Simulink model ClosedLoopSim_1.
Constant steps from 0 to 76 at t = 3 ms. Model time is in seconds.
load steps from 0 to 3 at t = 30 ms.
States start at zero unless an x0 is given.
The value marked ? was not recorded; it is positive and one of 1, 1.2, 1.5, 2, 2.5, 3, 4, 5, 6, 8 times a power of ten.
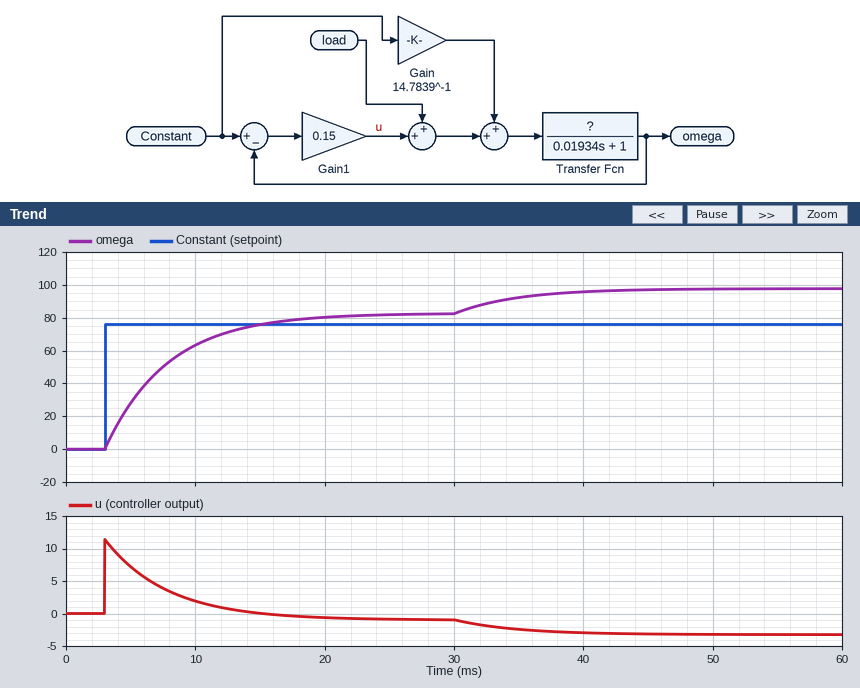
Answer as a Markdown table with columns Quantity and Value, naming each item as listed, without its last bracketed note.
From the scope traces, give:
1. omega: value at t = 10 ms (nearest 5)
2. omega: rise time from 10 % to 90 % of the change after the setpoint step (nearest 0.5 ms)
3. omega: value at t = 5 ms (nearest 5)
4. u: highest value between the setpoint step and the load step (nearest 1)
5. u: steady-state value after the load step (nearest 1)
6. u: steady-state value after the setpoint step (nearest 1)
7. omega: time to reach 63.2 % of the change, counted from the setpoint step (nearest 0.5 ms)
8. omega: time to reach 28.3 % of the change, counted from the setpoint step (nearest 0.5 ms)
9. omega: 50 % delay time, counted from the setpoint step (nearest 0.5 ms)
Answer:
| Quantity | Value |
|---|---|
| omega: value at t = 10 ms | 65 |
| omega: rise time from 10 % to 90 % of the change after the setpoint step | 10.5 ms |
| omega: value at t = 5 ms | 30 |
| u: highest value between the setpoint step and the load step | 11 |
| u: steady-state value after the load step | -3 |
| u: steady-state value after the setpoint step | -1 |
| omega: time to reach 63.2 % of the change, counted from the setpoint step | 5.0 ms |
| omega: time to reach 28.3 % of the change, counted from the setpoint step | 1.5 ms |
| omega: 50 % delay time, counted from the setpoint step | 3.5 ms |
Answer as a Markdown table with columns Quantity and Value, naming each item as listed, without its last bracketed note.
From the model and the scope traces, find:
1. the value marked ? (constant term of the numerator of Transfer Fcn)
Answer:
| Quantity | Value |
|---|---|
| the value marked ? | 20 |
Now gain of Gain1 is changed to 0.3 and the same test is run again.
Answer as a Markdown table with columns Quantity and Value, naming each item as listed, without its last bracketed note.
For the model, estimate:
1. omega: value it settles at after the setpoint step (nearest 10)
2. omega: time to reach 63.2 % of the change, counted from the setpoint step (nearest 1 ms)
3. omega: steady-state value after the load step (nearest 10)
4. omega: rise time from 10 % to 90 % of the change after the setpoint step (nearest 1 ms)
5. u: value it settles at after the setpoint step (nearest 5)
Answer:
| Quantity | Value |
|---|---|
| omega: value it settles at after the setpoint step | 80 |
| omega: time to reach 63.2 % of the change, counted from the setpoint step | 3 ms |
| omega: steady-state value after the load step | 90 |
| omega: rise time from 10 % to 90 % of the change after the setpoint step | 6 ms |
| u: value it settles at after the setpoint step | 0 |
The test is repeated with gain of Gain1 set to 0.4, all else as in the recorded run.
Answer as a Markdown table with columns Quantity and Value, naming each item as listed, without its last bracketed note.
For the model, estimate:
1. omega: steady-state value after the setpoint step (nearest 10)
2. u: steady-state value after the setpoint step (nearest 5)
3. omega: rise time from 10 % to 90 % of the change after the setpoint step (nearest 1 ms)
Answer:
| Quantity | Value |
|---|---|
| omega: steady-state value after the setpoint step | 80 |
| u: steady-state value after the setpoint step | 0 |
| omega: rise time from 10 % to 90 % of the change after the setpoint step | 5 ms |
